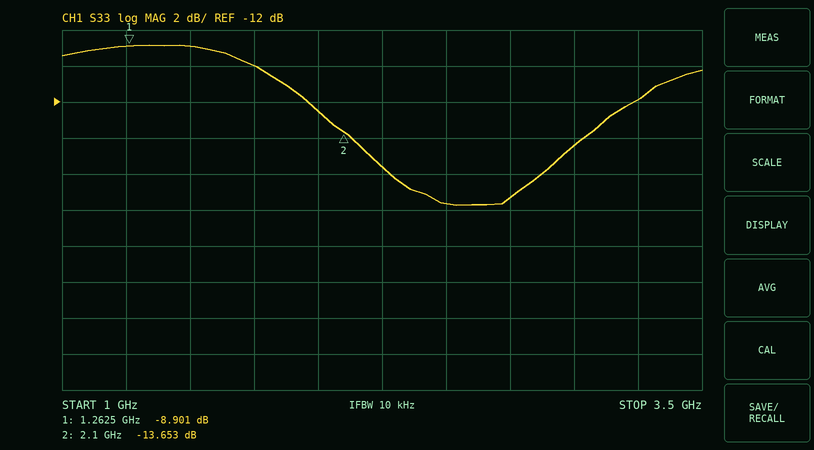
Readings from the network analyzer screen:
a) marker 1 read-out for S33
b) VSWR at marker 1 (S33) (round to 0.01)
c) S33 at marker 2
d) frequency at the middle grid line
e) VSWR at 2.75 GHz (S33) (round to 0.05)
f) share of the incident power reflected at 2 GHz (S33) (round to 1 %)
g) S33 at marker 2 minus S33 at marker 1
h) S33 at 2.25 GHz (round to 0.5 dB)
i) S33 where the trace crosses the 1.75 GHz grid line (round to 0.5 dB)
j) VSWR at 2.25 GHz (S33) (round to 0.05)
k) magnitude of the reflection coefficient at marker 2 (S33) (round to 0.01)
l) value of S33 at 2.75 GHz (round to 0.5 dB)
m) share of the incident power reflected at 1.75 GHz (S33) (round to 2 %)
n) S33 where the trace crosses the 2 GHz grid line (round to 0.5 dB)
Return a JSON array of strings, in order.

["-8.901 dB", "2.12", "-13.653 dB", "2.25 GHz", "1.30", "6 %", "-4.752 dB", "-15.5 dB", "-10.0 dB", "1.40", "0.21", "-17.5 dB", "10 %", "-12.5 dB"]
